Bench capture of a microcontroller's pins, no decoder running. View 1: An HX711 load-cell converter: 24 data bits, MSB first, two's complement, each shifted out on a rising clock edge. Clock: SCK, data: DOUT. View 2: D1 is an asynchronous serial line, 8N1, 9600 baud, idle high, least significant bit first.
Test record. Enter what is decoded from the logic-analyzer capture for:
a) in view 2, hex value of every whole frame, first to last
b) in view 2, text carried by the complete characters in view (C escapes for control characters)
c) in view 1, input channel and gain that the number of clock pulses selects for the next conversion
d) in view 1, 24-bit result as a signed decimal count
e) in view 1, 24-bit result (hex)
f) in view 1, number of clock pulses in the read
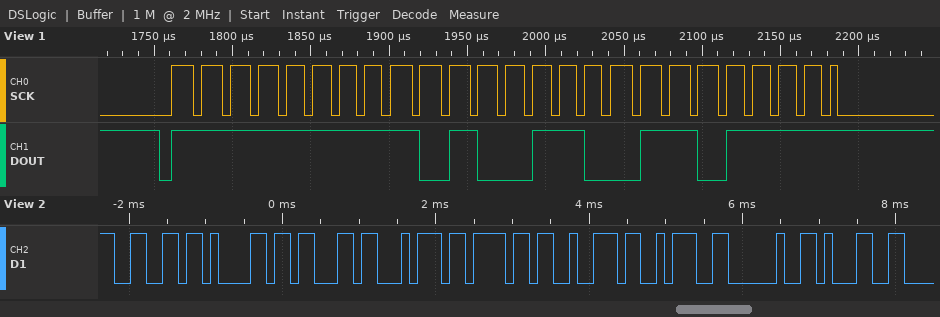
0x66 0x61 0x63 0x74 0x6F 0x72 0x3A 0x20 0x31
"factor: 1"
channel A, gain 128
-22929
0xFFA66F
25
